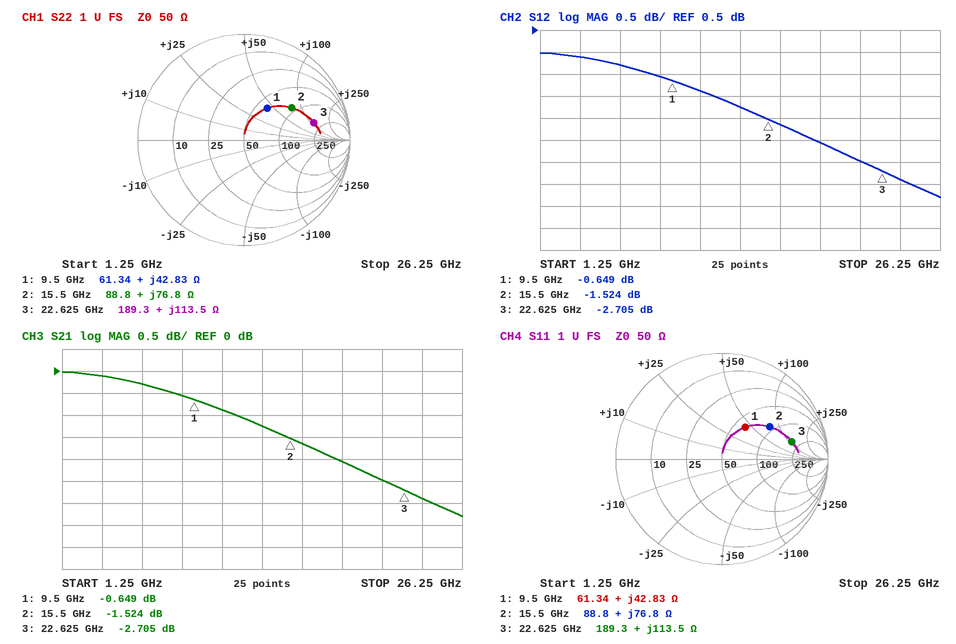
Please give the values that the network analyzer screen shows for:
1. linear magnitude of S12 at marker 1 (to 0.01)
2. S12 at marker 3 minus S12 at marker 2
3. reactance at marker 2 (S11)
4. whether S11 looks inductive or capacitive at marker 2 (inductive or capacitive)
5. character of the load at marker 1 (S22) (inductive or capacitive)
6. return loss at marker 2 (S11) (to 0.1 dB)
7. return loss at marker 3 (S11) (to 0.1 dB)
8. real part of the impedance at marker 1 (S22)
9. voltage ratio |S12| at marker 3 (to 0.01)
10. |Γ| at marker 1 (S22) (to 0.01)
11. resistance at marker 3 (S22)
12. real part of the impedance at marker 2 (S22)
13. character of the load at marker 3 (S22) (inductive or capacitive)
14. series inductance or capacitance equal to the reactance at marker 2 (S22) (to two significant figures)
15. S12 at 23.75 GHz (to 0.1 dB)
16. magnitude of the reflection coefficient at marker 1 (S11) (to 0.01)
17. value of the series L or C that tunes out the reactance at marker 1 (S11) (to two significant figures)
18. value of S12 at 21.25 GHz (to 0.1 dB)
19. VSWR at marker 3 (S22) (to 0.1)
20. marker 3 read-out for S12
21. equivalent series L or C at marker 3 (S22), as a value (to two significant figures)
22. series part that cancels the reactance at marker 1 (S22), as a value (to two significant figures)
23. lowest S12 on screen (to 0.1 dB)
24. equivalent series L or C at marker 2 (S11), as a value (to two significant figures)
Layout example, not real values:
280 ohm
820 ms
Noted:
0.93
-1.181 dB
+76.8 Ω
inductive
inductive
5.3 dB
3.4 dB
61.34 Ω
0.73
0.37
189.3 Ω
88.8 Ω
inductive
790 pH
-2.9 dB
0.37
390 fF
-2.5 dB
5.2
-2.705 dB
800 pH
390 fF
-3.3 dB
790 pH
